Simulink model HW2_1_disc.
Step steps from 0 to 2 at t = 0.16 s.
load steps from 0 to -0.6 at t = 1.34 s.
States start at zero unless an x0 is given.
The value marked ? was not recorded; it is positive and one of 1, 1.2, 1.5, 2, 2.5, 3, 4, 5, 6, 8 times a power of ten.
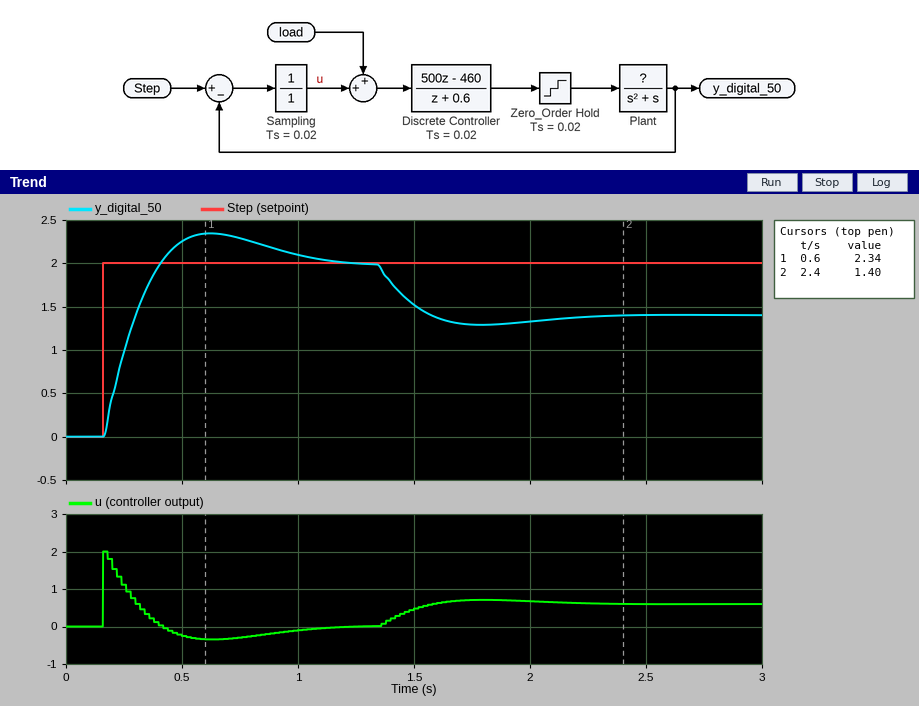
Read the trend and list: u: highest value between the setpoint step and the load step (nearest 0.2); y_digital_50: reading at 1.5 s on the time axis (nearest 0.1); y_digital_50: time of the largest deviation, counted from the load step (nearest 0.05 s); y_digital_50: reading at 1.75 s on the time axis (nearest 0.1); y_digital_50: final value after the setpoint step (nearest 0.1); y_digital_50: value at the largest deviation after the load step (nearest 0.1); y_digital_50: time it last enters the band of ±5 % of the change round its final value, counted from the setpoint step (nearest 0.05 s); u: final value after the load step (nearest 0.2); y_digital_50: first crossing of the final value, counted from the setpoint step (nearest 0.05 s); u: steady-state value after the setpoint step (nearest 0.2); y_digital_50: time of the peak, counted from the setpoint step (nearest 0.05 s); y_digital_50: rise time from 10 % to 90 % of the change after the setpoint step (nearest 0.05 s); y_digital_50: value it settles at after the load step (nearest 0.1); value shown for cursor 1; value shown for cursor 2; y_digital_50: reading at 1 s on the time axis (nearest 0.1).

2.0
1.5
0.45 s
1.3
2.0
1.3
0.85 s
0.6
0.25 s
0.0
0.45 s
0.20 s
1.4
2.34
1.40
2.1
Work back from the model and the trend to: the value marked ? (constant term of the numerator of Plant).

1
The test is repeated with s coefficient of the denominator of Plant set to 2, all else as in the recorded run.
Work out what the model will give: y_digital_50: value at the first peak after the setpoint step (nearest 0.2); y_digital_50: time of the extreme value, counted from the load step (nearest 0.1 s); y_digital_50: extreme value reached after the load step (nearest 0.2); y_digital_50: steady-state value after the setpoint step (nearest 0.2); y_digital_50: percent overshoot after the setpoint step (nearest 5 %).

2.2
0.5 s
1.4
2.0
10 %
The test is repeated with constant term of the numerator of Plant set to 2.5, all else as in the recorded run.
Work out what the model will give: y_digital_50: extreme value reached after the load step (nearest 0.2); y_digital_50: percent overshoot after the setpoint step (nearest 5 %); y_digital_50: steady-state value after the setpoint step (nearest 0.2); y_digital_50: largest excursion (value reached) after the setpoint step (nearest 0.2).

1.4
10 %
2.0
2.2
